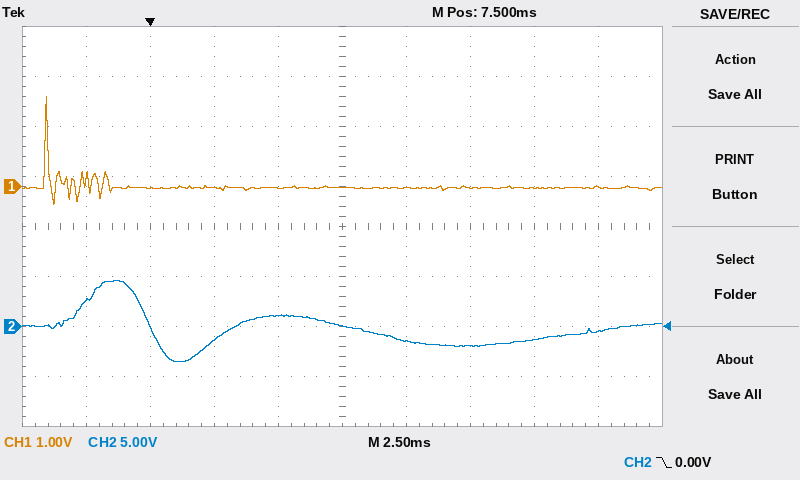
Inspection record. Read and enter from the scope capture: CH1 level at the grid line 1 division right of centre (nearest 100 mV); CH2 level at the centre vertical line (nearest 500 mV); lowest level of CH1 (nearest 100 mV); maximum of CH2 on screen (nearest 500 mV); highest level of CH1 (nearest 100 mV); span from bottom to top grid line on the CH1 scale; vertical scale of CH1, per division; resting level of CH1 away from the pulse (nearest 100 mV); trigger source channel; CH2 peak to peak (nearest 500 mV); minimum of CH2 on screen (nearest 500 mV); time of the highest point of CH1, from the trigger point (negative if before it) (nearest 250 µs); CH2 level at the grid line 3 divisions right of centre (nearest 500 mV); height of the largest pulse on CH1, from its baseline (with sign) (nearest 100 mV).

0.0 V
0.0 V
-400 mV
4.5 V
1.8 V
8 V
1 V
0.0 V
CH2
8.0 V
-3.5 V
-4.00 ms
-1.5 V
+1.8 V
